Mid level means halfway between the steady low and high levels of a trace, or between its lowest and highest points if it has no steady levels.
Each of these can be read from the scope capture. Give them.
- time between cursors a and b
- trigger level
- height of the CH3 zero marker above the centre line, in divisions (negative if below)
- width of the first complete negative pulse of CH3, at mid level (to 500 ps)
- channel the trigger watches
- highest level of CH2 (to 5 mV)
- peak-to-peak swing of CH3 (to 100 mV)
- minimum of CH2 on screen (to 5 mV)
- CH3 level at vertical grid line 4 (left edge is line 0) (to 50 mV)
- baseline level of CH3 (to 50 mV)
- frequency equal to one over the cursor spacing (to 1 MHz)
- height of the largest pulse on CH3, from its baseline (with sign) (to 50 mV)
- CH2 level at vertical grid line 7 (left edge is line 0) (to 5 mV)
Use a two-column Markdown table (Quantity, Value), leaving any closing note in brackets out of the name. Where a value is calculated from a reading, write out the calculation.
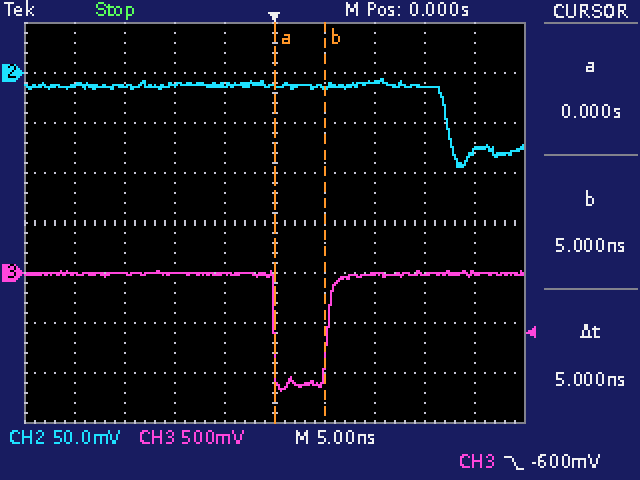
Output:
| Quantity | Value |
|---|---|
| time between cursors a and b | 5 ns |
| trigger level | -600 mV |
| height of the CH3 zero marker above the centre line, in divisions | -1.0 div |
| width of the first complete negative pulse of CH3, at mid level | 5.5 ns |
| channel the trigger watches | CH3 |
| highest level of CH2 | -5 mV |
| peak-to-peak swing of CH3 | 1.20 V |
| minimum of CH2 on screen | -95 mV |
| CH3 level at vertical grid line 4 (left edge is line 0) | 0 mV |
| baseline level of CH3 | 0 mV |
| frequency equal to one over the cursor spacing | 1 / 5 ns ≈ 200 MHz |
| height of the largest pulse on CH3, from its baseline (with sign) | -1.15 V |
| CH2 level at vertical grid line 7 (left edge is line 0) | -10 mV |
